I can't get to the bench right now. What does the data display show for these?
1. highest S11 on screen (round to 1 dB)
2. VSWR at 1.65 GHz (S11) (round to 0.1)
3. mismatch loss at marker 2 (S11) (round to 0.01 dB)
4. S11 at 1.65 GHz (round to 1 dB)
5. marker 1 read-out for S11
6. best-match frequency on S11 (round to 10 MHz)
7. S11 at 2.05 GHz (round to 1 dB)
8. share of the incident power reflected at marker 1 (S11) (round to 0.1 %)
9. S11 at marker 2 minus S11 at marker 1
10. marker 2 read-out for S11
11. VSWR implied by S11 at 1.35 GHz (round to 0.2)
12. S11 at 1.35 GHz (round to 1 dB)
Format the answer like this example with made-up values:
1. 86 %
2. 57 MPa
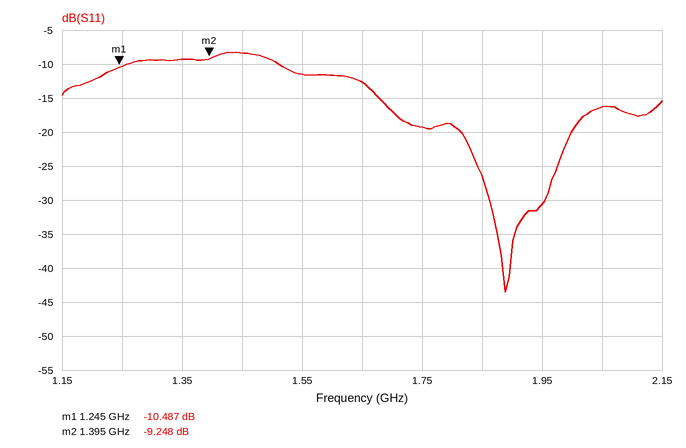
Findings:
1. -8 dB
2. 1.6
3. 0.55 dB
4. -13 dB
5. -10.487 dB
6. 1.89 GHz
7. -16 dB
8. 8.9 %
9. 1.239 dB
10. -9.248 dB
11. 2.0
12. -9 dB
